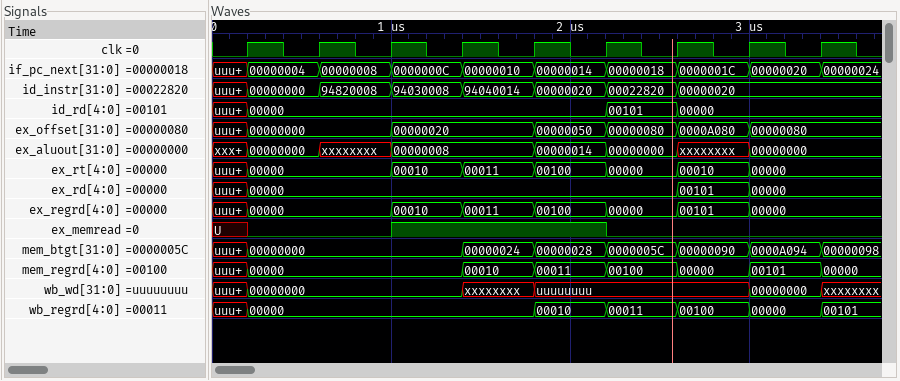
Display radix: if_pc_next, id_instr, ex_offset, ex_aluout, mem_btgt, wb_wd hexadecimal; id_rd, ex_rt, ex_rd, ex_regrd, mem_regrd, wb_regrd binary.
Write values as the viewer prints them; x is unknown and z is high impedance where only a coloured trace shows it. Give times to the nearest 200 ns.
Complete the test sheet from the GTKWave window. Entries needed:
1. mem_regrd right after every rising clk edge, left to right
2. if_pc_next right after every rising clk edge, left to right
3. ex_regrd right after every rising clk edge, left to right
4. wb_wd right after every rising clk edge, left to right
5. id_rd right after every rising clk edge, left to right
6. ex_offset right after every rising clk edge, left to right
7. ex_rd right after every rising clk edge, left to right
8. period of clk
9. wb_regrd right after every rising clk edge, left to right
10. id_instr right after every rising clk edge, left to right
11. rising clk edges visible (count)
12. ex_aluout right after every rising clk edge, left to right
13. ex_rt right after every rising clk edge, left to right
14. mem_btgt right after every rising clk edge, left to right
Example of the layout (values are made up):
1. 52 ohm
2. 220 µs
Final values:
1. 00000, 00000, 00000, 00010, 00011, 00100, 00000, 00101, 00000
2. 00000004, 00000008, 0000000C, 00000010, 00000014, 00000018, 0000001C, 00000020, 00000024
3. 00000, 00000, 00010, 00011, 00100, 00000, 00101, 00000, 00000
4. 00000000, 00000000, 00000000, xxxxxxxx, uuuuuuuu, uuuuuuuu, uuuuuuuu, 00000000, xxxxxxxx
5. 00000, 00000, 00000, 00000, 00000, 00101, 00000, 00000, 00000
6. 00000000, 00000000, 00000020, 00000020, 00000050, 00000080, 0000A080, 00000080, 00000080
7. 00000, 00000, 00000, 00000, 00000, 00000, 00101, 00000, 00000
8. 400 ns
9. 00000, 00000, 00000, 00000, 00010, 00011, 00100, 00000, 00101
10. 00000000, 94820008, 94030008, 94040014, 00000020, 00022820, 00000020, 00000020, 00000020
11. 9
12. 00000000, xxxxxxxx, 00000008, 00000008, 00000014, 00000000, xxxxxxxx, 00000000, 00000000
13. 00000, 00000, 00010, 00011, 00100, 00000, 00010, 00000, 00000
14. 00000000, 00000000, 00000000, 00000024, 00000028, 0000005C, 00000090, 0000A094, 00000098
